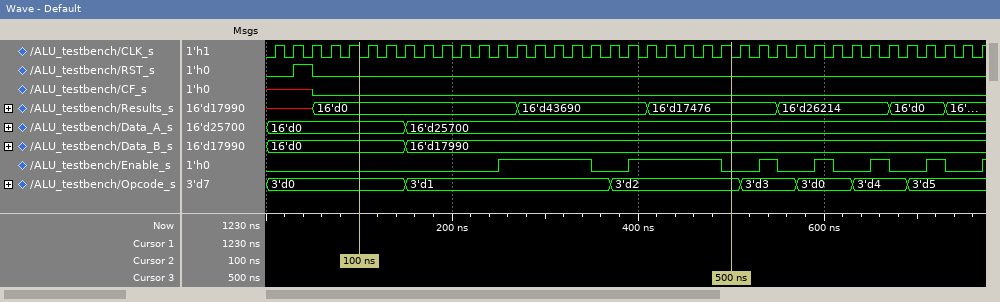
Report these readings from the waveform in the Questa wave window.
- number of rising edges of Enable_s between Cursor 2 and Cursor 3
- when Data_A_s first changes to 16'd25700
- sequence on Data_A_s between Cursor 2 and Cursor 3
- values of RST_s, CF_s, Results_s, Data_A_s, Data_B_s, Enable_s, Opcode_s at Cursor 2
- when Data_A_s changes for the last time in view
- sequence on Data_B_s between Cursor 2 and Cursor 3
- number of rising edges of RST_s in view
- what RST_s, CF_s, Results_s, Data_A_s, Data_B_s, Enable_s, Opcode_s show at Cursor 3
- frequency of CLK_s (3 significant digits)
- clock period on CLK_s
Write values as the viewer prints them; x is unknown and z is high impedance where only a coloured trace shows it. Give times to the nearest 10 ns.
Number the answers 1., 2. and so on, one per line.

1. 2
2. 150 ns
3. 16'd0, 16'd25700
4. RST_s=0, CF_s=0, Results_s=16'd0, Data_A_s=16'd0, Data_B_s=16'd0, Enable_s=0, Opcode_s=3'd0
5. 150 ns
6. 16'd0, 16'd17990
7. 1
8. RST_s=0, CF_s=0, Results_s=16'd17476, Data_A_s=16'd25700, Data_B_s=16'd17990, Enable_s=0, Opcode_s=3'd2
9. 50.0 MHz
10. 20 ns
